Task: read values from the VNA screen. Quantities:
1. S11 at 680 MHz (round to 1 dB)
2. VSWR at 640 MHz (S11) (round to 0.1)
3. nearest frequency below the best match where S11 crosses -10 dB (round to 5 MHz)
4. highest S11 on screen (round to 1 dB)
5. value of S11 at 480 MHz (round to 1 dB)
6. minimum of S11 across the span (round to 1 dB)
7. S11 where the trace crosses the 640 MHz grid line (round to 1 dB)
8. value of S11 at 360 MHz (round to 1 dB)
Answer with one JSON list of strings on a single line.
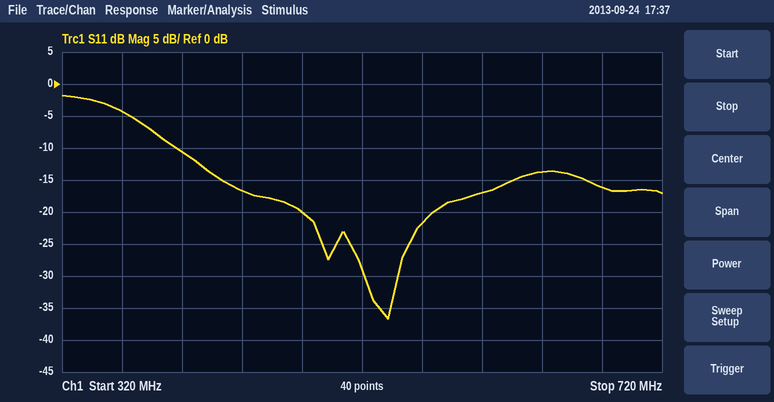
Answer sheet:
["-16 dB", "1.5", "395 MHz", "-2 dB", "-20 dB", "-37 dB", "-14 dB", "-4 dB"]
